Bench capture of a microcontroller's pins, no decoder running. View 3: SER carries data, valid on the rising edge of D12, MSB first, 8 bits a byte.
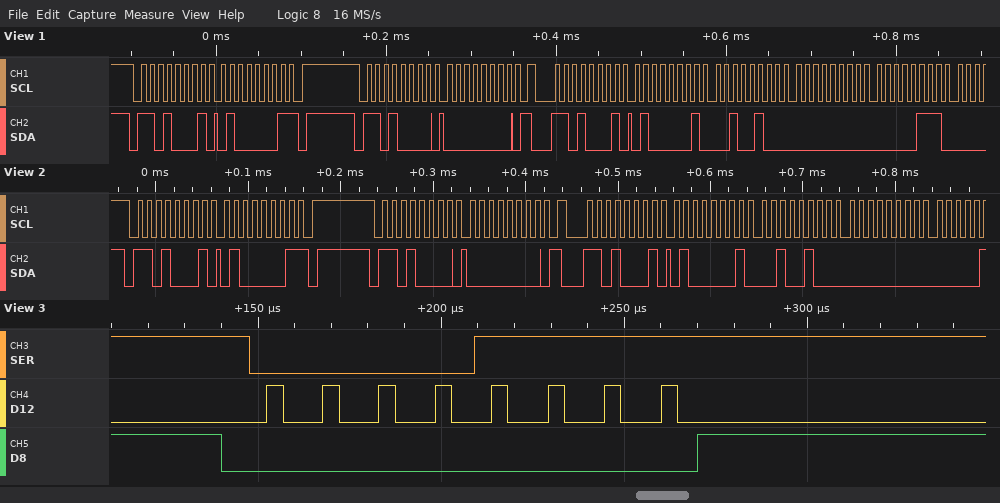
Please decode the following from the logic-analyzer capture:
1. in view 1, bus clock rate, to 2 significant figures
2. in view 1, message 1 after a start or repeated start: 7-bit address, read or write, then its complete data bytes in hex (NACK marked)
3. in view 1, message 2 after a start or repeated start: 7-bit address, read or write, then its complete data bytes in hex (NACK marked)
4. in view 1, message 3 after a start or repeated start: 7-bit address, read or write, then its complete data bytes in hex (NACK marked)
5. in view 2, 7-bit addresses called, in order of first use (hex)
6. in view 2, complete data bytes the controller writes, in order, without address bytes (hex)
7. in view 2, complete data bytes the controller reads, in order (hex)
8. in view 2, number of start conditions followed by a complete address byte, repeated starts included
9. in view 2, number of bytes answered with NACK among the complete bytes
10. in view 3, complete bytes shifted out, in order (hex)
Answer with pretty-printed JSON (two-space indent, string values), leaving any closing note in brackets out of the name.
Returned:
{
  "in view 1, bus clock rate, to 2 significant figures": "100 kHz",
  "in view 1, message 1 after a start or repeated start: 7-bit address, read or write, then its complete data bytes in hex": "0x68 read: 41 NACK",
  "in view 1, message 2 after a start or repeated start: 7-bit address, read or write, then its complete data bytes in hex": "0x68 write: 00",
  "in view 1, message 3 after a start or repeated start: 7-bit address, read or write, then its complete data bytes in hex": "0x68 read: 41 24 00 07",
  "in view 2, 7-bit addresses called, in order of first use": "0x68",
  "in view 2, complete data bytes the controller writes, in order, without address bytes": "00",
  "in view 2, complete data bytes the controller reads, in order": "41 41 24 00",
  "in view 2, number of start conditions followed by a complete address byte, repeated starts included": "3",
  "in view 2, number of bytes answered with NACK among the complete bytes": "1",
  "in view 3, complete bytes shifted out, in order": "0x0F"
}
